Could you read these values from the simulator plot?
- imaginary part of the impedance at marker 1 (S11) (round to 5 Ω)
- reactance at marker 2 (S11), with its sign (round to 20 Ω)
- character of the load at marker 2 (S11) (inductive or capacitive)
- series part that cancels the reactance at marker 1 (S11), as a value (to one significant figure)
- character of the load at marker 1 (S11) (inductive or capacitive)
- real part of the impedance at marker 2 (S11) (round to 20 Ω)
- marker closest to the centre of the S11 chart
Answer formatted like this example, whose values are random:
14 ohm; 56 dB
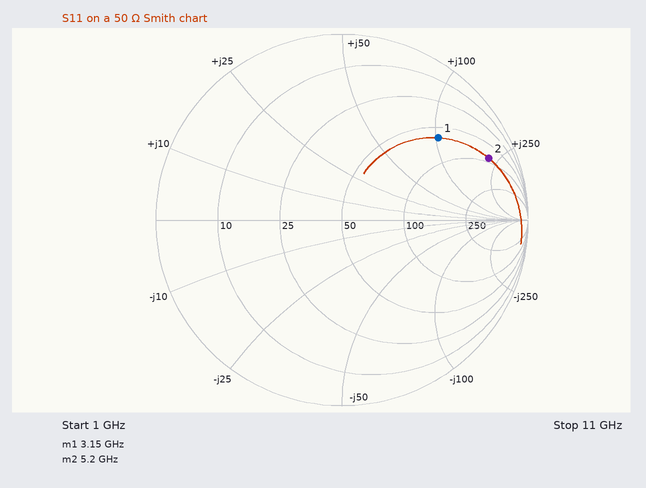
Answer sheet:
+105 Ω; +220 Ω; inductive; 500 fF; inductive; 80 Ω; marker 1
